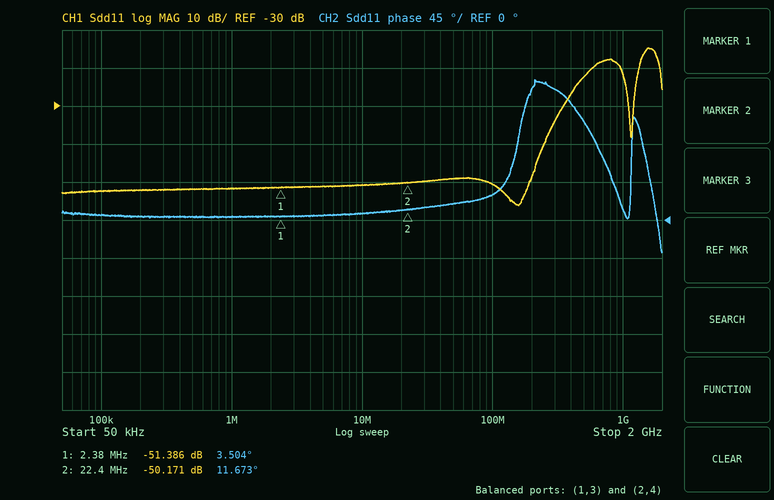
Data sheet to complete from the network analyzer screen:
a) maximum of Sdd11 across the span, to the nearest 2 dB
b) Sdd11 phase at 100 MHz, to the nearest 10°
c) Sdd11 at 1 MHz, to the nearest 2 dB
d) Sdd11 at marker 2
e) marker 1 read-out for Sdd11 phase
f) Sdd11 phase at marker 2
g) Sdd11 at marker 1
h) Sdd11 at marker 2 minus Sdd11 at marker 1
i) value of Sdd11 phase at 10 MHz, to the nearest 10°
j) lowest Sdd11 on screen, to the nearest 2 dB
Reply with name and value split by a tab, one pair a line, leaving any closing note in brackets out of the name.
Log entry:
maximum of Sdd11 across the span, to the nearest 2 dB	-14 dB
Sdd11 phase at 100 MHz, to the nearest 10°	30°
Sdd11 at 1 MHz, to the nearest 2 dB	-52 dB
Sdd11 at marker 2	-50.171 dB
marker 1 read-out for Sdd11 phase	3.504°
Sdd11 phase at marker 2	11.673°
Sdd11 at marker 1	-51.386 dB
Sdd11 at marker 2 minus Sdd11 at marker 1	1.215 dB
value of Sdd11 phase at 10 MHz, to the nearest 10°	10°
lowest Sdd11 on screen, to the nearest 2 dB	-56 dB
